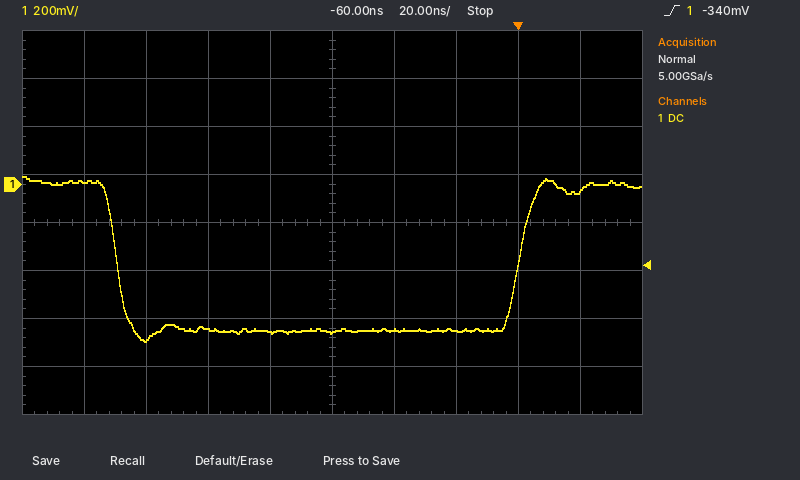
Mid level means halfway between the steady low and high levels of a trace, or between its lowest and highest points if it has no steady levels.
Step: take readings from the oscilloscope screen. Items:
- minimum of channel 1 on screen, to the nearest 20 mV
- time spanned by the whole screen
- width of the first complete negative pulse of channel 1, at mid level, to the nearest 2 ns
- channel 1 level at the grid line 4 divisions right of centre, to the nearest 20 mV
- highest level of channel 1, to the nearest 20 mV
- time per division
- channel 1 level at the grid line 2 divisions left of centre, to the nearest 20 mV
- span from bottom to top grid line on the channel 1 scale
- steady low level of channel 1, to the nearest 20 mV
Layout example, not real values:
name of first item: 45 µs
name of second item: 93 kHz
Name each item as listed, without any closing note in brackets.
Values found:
minimum of channel 1 on screen, to the nearest 20 mV: -660 mV
time spanned by the whole screen: 200 ns
width of the first complete negative pulse of channel 1, at mid level, to the nearest 2 ns: 130 ns
channel 1 level at the grid line 4 divisions right of centre, to the nearest 20 mV: -20 mV
highest level of channel 1, to the nearest 20 mV: 40 mV
time per division: 20 ns
channel 1 level at the grid line 2 divisions left of centre, to the nearest 20 mV: -600 mV
span from bottom to top grid line on the channel 1 scale: 1.6 V
steady low level of channel 1, to the nearest 20 mV: -600 mV
